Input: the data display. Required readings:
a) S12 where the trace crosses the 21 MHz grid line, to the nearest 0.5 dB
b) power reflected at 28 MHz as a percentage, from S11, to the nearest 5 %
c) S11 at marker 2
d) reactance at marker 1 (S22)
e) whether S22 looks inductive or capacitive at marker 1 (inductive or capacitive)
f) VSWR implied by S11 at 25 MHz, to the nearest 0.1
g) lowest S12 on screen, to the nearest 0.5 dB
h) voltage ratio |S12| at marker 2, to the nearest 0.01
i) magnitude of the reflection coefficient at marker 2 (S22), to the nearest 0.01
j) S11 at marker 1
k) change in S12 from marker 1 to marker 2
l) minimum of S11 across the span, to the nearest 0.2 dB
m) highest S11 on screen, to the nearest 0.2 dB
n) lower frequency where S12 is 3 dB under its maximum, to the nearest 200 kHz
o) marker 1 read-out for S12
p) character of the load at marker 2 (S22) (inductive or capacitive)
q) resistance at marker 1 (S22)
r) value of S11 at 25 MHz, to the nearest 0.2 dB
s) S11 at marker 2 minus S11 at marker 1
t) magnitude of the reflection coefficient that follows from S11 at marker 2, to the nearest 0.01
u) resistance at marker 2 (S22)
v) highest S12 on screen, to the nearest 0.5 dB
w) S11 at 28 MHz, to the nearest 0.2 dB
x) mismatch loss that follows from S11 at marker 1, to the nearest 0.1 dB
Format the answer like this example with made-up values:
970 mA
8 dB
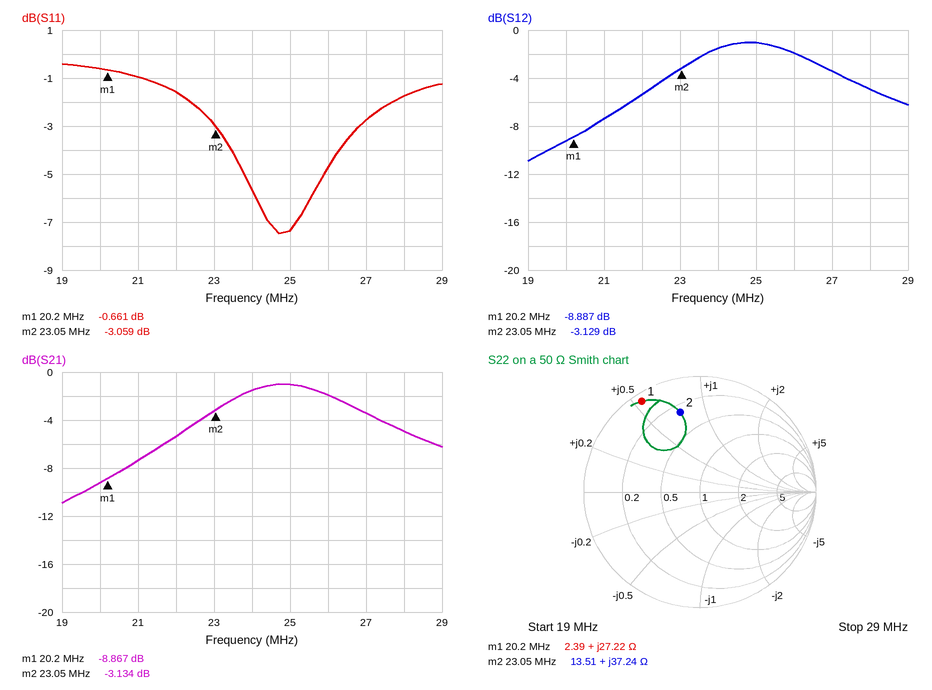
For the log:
-7.5 dB
65 %
-3.059 dB
+27.22 Ω
inductive
2.5
-11.0 dB
0.70
0.71
-0.661 dB
5.758 dB
-7.4 dB
-0.4 dB
22.6 MHz
-8.887 dB
inductive
2.39 Ω
-7.4 dB
-2.398 dB
0.70
13.51 Ω
-1.0 dB
-1.8 dB
8.5 dB
